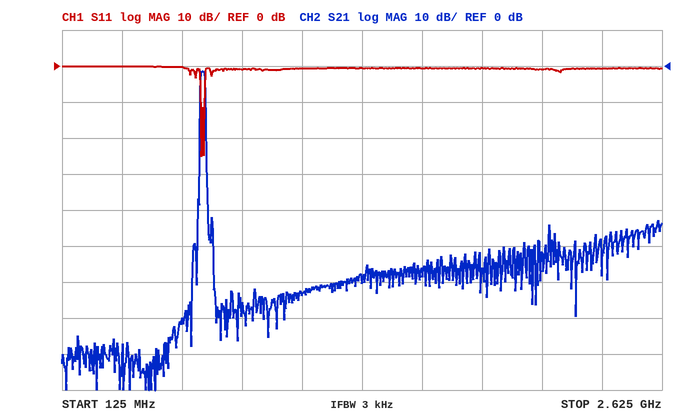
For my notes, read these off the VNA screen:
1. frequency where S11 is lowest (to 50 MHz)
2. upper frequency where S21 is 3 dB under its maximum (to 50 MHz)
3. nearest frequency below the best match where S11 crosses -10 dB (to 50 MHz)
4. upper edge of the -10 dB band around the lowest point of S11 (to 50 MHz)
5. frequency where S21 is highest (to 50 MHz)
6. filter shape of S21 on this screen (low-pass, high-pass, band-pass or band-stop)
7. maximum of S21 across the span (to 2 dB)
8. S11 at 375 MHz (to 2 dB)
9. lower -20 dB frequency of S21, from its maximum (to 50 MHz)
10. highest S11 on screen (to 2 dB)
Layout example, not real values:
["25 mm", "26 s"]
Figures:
["700 MHz", "700 MHz", "700 MHz", "700 MHz", "700 MHz", "band-pass", "-2 dB", "0 dB", "700 MHz", "0 dB"]
